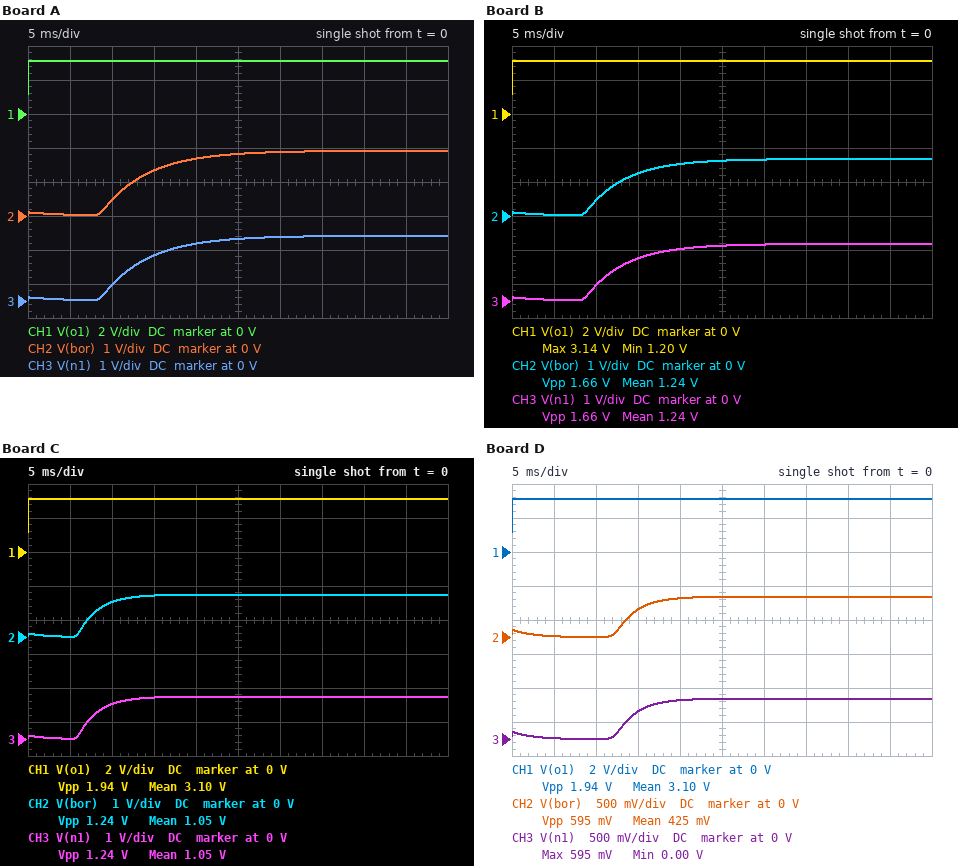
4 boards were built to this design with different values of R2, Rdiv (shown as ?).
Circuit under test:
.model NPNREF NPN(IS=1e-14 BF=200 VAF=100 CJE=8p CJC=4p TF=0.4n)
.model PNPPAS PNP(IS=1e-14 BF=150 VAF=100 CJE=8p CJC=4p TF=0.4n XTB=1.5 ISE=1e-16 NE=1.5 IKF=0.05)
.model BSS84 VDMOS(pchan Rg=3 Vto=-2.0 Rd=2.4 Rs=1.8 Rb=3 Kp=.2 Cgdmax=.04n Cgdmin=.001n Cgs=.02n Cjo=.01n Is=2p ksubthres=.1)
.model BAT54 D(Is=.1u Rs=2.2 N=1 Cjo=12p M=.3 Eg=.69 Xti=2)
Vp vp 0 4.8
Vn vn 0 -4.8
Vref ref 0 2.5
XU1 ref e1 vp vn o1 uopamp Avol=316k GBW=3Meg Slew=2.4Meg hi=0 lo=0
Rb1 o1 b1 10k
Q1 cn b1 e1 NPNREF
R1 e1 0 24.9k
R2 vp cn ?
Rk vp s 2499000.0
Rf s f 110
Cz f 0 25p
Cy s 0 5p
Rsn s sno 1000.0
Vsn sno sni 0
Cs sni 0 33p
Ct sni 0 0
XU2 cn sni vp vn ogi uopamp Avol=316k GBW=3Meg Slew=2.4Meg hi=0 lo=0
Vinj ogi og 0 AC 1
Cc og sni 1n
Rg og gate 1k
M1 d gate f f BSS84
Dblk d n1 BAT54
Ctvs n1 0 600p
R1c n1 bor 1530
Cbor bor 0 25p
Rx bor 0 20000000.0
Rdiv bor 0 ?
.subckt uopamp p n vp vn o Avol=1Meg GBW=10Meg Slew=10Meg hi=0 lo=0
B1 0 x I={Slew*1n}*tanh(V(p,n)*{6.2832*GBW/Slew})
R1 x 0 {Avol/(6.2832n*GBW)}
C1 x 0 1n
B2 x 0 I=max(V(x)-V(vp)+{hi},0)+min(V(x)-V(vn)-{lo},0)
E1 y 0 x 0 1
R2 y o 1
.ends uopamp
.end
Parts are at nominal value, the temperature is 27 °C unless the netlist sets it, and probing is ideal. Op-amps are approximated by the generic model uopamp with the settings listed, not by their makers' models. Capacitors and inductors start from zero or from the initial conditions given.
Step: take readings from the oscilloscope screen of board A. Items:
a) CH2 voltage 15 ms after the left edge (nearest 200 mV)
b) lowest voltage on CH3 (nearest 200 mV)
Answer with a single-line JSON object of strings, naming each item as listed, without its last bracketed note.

{"CH2 voltage 15 ms after the left edge": "1.4 V", "lowest voltage on CH3": "0 V"}
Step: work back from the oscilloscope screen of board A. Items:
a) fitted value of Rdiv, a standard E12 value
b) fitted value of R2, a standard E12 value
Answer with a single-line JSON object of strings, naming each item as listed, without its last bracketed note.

{"fitted value of Rdiv, a standard E12 value": "15 MΩ", "fitted value of R2, a standard E12 value": "5.6 kΩ"}
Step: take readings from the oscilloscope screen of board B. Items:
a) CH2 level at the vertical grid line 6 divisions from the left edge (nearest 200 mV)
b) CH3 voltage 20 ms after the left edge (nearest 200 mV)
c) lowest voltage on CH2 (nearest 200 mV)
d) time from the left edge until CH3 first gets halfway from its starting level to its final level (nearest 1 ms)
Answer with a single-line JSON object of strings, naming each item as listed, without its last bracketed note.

{"CH2 level at the vertical grid line 6 divisions from the left edge": "1.6 V", "CH3 voltage 20 ms after the left edge": "1.6 V", "lowest voltage on CH2": "0 V", "time from the left edge until CH3 first gets halfway from its starting level to its final level": "12 ms"}
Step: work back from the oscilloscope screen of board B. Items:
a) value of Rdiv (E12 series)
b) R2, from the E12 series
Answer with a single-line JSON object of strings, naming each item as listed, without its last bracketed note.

{"value of Rdiv": "12 MΩ", "R2, from the E12 series": "5.6 kΩ"}
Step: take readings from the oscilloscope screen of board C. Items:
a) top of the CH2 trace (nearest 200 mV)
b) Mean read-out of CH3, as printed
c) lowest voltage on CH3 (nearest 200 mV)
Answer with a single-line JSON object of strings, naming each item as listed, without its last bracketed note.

{"top of the CH2 trace": "1.2 V", "Mean read-out of CH3, as printed": "1.05 V", "lowest voltage on CH3": "0 V"}
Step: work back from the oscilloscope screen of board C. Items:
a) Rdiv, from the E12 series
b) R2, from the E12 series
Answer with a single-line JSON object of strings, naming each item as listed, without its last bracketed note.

{"Rdiv, from the E12 series": "4.7 MΩ", "R2, from the E12 series": "8.2 kΩ"}
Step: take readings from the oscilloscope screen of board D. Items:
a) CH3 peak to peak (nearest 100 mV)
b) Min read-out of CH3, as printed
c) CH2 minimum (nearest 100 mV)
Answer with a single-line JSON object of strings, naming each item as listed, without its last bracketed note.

{"CH3 peak to peak": "600 mV", "Min read-out of CH3, as printed": "0.00 V", "CH2 minimum": "0 V"}
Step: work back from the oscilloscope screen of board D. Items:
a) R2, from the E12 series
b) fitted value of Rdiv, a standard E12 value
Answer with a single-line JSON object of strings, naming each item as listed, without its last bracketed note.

{"R2, from the E12 series": "3.9 kΩ", "fitted value of Rdiv, a standard E12 value": "4.7 MΩ"}
